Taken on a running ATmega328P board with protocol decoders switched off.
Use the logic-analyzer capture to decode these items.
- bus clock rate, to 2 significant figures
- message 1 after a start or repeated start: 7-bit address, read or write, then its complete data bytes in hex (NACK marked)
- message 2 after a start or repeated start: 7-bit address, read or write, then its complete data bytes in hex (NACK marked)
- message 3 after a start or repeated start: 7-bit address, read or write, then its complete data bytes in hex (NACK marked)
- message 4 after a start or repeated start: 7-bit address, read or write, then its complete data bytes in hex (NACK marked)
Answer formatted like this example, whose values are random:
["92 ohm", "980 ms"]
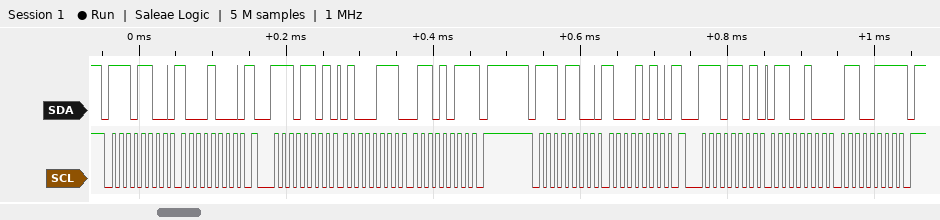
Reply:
["100 kHz", "0x76 write: 88", "0x76 read: 47 6B NACK", "0x76 write: 8A", "0x76 read: 64 67 NACK"]
